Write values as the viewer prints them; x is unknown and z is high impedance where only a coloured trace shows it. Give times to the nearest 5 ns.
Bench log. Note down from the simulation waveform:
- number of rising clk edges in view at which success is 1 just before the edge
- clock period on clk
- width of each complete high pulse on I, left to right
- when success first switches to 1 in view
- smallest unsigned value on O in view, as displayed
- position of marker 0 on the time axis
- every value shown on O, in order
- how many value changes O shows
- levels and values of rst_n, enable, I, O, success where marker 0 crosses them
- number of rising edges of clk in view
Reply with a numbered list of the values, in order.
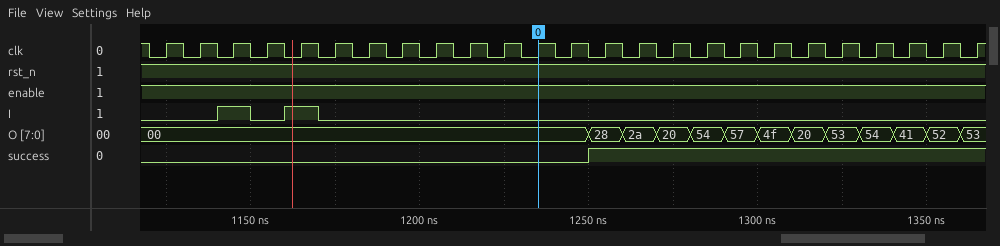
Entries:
1. 12
2. 10 ns
3. 10 ns, 10 ns
4. 1250 ns
5. 00
6. 1235 ns
7. 00, 28, 2a, 20, 54, 57, 4f, 20, 53, 54, 41, 52, 53
8. 12
9. rst_n=1, enable=1, I=0, O=00, success=0
10. 25
